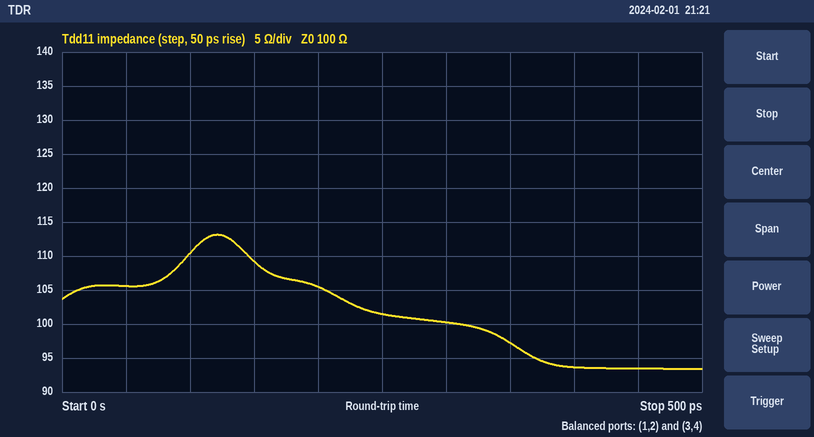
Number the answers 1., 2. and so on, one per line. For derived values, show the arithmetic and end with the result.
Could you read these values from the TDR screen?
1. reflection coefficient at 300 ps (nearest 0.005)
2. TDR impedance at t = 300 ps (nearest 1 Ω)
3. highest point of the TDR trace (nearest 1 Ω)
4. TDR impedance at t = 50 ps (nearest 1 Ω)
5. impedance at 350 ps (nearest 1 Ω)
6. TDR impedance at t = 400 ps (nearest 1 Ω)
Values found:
1. (100 − 100)/(100 + 100) ≈ 0.000
2. 100 Ω
3. 113 Ω
4. 106 Ω
5. 97 Ω
6. 94 Ω
